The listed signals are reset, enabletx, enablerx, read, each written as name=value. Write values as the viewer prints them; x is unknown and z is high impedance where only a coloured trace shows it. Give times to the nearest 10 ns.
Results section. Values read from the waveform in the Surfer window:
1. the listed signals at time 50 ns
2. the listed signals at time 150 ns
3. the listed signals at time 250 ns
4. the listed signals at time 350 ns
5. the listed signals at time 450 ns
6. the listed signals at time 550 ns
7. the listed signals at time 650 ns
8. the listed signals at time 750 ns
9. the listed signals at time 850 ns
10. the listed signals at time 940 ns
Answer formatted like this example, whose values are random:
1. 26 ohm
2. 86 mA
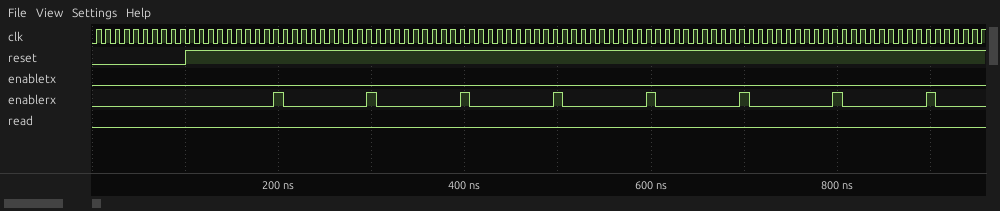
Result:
1. reset=0, enabletx=0, enablerx=0, read=0
2. reset=1, enabletx=0, enablerx=0, read=0
3. reset=1, enabletx=0, enablerx=0, read=0
4. reset=1, enabletx=0, enablerx=0, read=0
5. reset=1, enabletx=0, enablerx=0, read=0
6. reset=1, enabletx=0, enablerx=0, read=0
7. reset=1, enabletx=0, enablerx=0, read=0
8. reset=1, enabletx=0, enablerx=0, read=0
9. reset=1, enabletx=0, enablerx=0, read=0
10. reset=1, enabletx=0, enablerx=0, read=0
